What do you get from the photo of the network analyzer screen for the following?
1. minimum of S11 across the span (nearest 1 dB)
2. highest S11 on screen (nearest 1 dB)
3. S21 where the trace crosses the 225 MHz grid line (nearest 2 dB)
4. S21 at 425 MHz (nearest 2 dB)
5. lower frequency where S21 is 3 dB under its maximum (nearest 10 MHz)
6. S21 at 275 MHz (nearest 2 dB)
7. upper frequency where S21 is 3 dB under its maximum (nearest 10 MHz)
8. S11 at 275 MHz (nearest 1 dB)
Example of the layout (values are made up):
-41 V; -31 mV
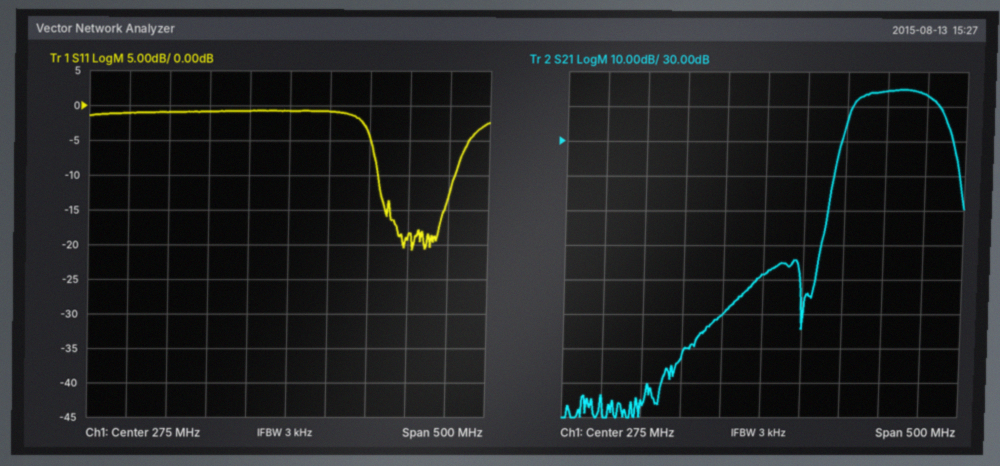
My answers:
-21 dB; -1 dB; -20 dB; 44 dB; 390 MHz; -8 dB; 480 MHz; -1 dB
